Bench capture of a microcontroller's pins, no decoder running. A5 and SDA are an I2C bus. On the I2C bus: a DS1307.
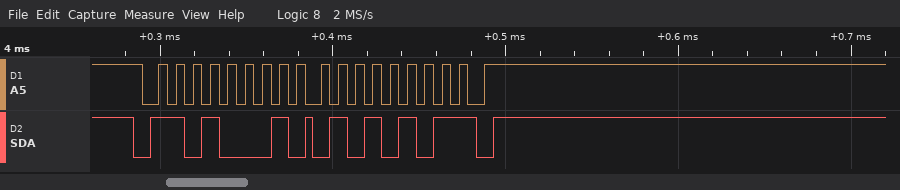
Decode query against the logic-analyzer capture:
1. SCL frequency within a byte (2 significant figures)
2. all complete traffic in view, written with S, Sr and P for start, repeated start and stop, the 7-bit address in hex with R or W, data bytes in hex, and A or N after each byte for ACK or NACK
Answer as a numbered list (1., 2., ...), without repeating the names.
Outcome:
1. 100 kHz
2. S 68R A 55 N P
